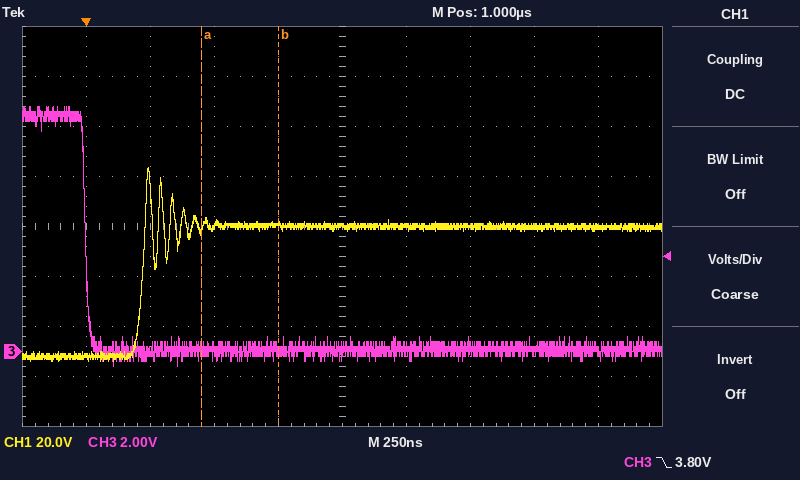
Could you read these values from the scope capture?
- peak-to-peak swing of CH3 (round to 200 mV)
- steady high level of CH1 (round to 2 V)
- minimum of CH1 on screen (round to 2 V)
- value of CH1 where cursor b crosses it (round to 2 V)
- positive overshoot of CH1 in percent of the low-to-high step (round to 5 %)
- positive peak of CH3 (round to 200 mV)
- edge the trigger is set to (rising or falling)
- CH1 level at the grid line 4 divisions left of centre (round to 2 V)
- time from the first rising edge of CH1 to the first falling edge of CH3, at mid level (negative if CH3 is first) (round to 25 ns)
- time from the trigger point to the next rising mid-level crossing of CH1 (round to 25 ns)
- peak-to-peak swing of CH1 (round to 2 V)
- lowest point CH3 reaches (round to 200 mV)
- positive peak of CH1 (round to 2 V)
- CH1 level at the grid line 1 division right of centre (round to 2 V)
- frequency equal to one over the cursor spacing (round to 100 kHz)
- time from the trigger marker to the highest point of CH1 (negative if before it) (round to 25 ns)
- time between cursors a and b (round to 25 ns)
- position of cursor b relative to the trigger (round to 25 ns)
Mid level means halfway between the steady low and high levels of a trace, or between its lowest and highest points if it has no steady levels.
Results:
10.4 V
50 V
-4 V
50 V
45 %
9.8 V
falling
-2 V
-225 ns
225 ns
78 V
-600 mV
74 V
50 V
3.3 MHz
+250 ns
300 ns
+750 ns
